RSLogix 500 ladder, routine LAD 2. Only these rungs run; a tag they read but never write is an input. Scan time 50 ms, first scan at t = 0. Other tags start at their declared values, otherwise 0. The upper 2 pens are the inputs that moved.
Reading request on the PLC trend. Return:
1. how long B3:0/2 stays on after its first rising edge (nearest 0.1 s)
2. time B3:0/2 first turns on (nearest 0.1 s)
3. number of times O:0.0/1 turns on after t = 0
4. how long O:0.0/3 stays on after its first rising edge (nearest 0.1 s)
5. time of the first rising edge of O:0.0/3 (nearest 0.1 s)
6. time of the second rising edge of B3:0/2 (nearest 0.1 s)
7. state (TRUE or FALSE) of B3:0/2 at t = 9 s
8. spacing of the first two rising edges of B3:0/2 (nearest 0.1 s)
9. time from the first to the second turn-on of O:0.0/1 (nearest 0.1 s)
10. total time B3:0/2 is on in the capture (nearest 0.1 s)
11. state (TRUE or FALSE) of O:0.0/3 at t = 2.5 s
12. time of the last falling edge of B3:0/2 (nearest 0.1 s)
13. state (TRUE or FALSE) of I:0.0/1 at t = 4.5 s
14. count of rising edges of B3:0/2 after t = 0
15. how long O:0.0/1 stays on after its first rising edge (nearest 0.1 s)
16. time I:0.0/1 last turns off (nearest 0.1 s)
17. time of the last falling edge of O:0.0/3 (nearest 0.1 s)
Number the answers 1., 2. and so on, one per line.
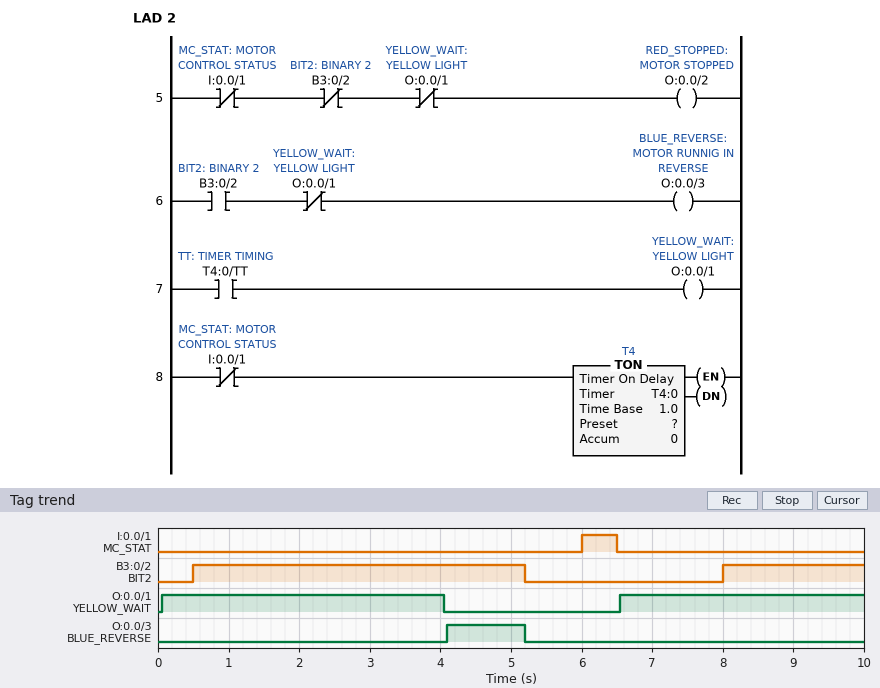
1. 4.7 s
2. 0.5 s
3. 2
4. 1.1 s
5. 4.1 s
6. 8.0 s
7. TRUE
8. 7.5 s
9. 6.5 s
10. 6.7 s
11. FALSE
12. 5.2 s
13. FALSE
14. 2
15. 4.0 s
16. 6.5 s
17. 5.2 s
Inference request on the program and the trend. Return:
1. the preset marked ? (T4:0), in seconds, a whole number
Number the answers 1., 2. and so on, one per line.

1. 4 s
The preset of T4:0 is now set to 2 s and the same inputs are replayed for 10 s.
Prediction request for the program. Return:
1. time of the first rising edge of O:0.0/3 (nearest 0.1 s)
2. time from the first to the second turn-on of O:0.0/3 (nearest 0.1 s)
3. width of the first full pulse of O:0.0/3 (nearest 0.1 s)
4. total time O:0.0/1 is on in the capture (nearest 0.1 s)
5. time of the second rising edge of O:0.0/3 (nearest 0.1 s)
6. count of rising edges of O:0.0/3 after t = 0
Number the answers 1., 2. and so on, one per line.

1. 2.1 s
2. 6.5 s
3. 3.1 s
4. 4.0 s
5. 8.6 s
6. 2
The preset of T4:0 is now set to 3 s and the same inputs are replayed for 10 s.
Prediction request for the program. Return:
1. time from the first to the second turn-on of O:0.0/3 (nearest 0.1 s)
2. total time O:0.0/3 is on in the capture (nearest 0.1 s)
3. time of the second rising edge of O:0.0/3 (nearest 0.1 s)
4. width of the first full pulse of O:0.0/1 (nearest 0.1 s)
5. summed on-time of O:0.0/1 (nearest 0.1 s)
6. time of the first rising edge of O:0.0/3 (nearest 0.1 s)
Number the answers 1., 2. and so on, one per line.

1. 6.5 s
2. 2.5 s
3. 9.6 s
4. 3.0 s
5. 6.0 s
6. 3.1 s
